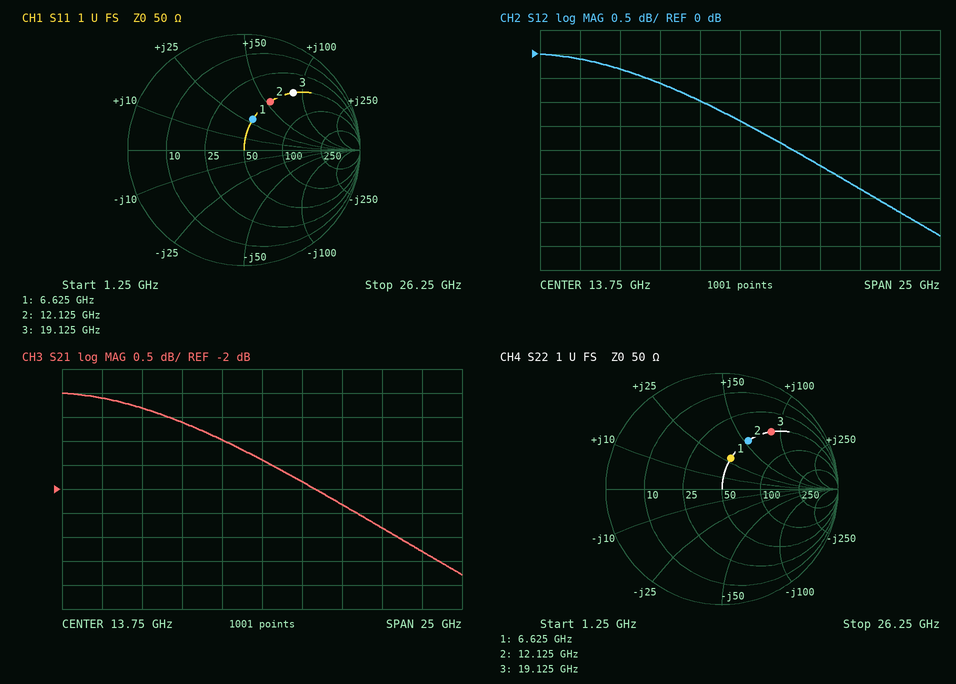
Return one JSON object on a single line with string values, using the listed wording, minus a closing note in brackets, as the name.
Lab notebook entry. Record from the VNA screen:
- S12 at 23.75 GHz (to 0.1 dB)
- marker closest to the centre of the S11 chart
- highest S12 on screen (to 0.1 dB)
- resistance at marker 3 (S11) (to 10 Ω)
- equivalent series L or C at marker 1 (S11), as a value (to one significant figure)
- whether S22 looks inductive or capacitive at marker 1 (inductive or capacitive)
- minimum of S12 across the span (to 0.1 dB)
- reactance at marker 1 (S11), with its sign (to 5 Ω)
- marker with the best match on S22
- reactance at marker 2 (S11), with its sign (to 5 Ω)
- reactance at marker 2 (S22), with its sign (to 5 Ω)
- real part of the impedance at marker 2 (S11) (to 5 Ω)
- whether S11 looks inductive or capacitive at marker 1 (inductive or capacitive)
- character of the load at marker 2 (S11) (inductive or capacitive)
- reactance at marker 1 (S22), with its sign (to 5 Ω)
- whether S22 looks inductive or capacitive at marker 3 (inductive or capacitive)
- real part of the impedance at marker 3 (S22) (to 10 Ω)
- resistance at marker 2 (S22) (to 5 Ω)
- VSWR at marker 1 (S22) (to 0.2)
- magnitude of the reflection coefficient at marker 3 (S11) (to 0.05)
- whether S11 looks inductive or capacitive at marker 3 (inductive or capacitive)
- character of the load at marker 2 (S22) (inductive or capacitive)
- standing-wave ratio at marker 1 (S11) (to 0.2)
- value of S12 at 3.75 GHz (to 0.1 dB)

{"S12 at 23.75 GHz": "-3.3 dB", "marker closest to the centre of the S11 chart": "marker 1", "highest S12 on screen": "0.0 dB", "resistance at marker 3 (S11)": "50 Ω", "equivalent series L or C at marker 1 (S11), as a value": "700 pH", "whether S22 looks inductive or capacitive at marker 1": "inductive", "minimum of S12 across the span": "-3.8 dB", "reactance at marker 1 (S11), with its sign": "+30 Ω", "marker with the best match on S22": "marker 1", "reactance at marker 2 (S11), with its sign": "+55 Ω", "reactance at marker 2 (S22), with its sign": "+55 Ω", "real part of the impedance at marker 2 (S11)": "50 Ω", "whether S11 looks inductive or capacitive at marker 1": "inductive", "character of the load at marker 2 (S11)": "inductive", "reactance at marker 1 (S22), with its sign": "+30 Ω", "whether S22 looks inductive or capacitive at marker 3": "inductive", "real part of the impedance at marker 3 (S22)": "50 Ω", "resistance at marker 2 (S22)": "50 Ω", "VSWR at marker 1 (S22)": "1.8", "magnitude of the reflection coefficient at marker 3 (S11)": "0.65", "whether S11 looks inductive or capacitive at marker 3": "inductive", "character of the load at marker 2 (S22)": "inductive", "standing-wave ratio at marker 1 (S11)": "1.8", "value of S12 at 3.75 GHz": "-0.1 dB"}
